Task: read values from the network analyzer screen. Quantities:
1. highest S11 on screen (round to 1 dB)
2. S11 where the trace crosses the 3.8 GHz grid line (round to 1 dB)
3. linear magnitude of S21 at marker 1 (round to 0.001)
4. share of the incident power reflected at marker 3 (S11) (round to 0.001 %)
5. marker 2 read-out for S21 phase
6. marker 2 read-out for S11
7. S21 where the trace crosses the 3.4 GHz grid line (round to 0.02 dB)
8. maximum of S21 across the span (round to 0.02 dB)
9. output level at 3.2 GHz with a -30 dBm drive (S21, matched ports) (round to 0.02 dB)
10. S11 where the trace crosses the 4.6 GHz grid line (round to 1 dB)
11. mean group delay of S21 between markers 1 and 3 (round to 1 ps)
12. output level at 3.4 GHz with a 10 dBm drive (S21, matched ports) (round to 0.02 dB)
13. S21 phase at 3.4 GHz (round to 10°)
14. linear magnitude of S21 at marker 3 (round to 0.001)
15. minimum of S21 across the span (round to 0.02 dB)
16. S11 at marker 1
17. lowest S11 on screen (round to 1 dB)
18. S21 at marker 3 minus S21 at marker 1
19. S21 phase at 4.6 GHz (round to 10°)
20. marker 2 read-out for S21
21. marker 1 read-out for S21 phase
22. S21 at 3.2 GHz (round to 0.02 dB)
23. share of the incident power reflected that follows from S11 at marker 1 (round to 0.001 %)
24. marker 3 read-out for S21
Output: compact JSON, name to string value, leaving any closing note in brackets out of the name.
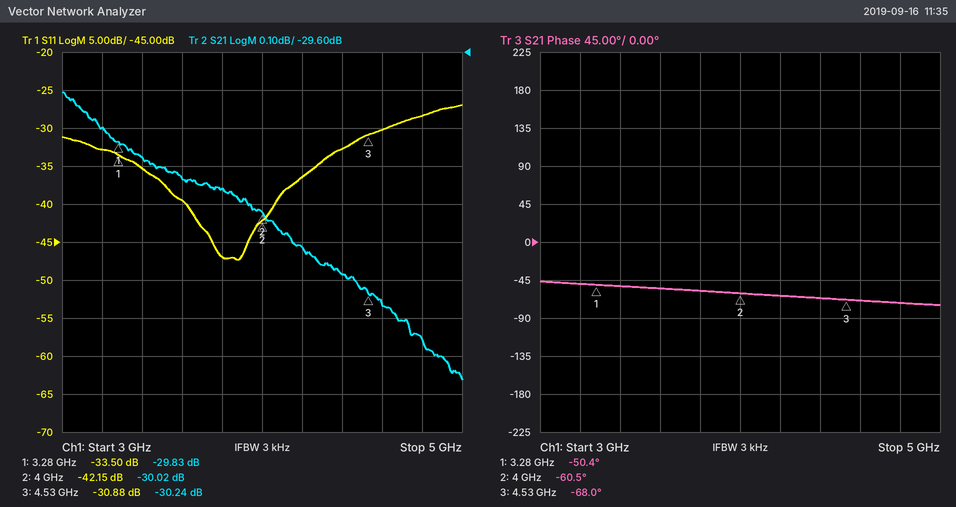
{"highest S11 on screen": "-27 dB", "S11 where the trace crosses the 3.8 GHz grid line": "-47 dB", "linear magnitude of S21 at marker 1": "0.032", "share of the incident power reflected at marker 3 (S11)": "0.082 %", "marker 2 read-out for S21 phase": "-60.5°", "marker 2 read-out for S11": "-42.15 dB", "S21 where the trace crosses the 3.4 GHz grid line": "-29.88 dB", "maximum of S21 across the span": "-29.70 dB", "output level at 3.2 GHz with a -30 dBm drive (S21, matched ports)": "-59.80 dBm", "S11 where the trace crosses the 4.6 GHz grid line": "-30 dB", "mean group delay of S21 between markers 1 and 3": "39 ps", "output level at 3.4 GHz with a 10 dBm drive (S21, matched ports)": "-19.88 dBm", "S21 phase at 3.4 GHz": "-50°", "linear magnitude of S21 at marker 3": "0.031", "minimum of S21 across the span": "-30.46 dB", "S11 at marker 1": "-33.50 dB", "lowest S11 on screen": "-47 dB", "S21 at marker 3 minus S21 at marker 1": "-0.41 dB", "S21 phase at 4.6 GHz": "-70°", "marker 2 read-out for S21": "-30.02 dB", "marker 1 read-out for S21 phase": "-50.4°", "S21 at 3.2 GHz": "-29.80 dB", "share of the incident power reflected that follows from S11 at marker 1": "0.045 %", "marker 3 read-out for S21": "-30.24 dB"}
